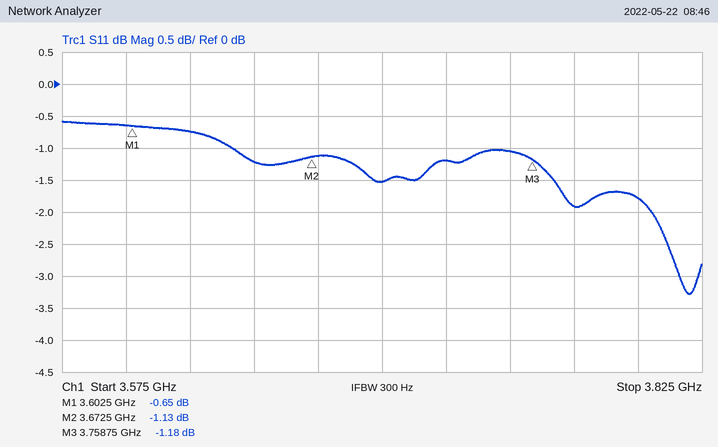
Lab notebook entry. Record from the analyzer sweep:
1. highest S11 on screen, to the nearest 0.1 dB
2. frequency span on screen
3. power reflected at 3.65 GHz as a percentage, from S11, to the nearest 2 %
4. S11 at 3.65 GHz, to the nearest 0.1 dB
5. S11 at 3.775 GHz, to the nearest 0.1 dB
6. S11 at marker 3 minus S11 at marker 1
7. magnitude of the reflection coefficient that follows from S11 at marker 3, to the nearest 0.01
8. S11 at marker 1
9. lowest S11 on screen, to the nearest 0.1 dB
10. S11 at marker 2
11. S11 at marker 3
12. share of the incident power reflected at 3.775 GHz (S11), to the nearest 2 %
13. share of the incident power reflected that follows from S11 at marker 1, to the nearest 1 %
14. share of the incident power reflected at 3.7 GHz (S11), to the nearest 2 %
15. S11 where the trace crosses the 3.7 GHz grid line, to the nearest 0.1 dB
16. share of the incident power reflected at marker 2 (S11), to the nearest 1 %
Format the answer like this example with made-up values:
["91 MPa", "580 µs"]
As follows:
["-0.6 dB", "250 MHz", "76 %", "-1.2 dB", "-1.9 dB", "-0.53 dB", "0.87", "-0.65 dB", "-3.3 dB", "-1.13 dB", "-1.18 dB", "64 %", "86 %", "70 %", "-1.5 dB", "77 %"]
